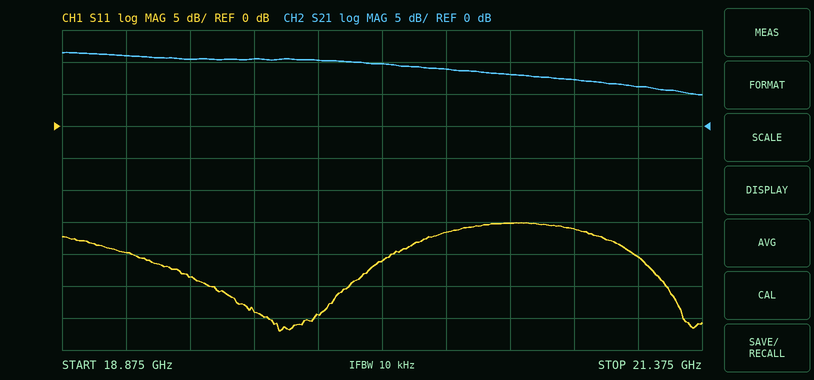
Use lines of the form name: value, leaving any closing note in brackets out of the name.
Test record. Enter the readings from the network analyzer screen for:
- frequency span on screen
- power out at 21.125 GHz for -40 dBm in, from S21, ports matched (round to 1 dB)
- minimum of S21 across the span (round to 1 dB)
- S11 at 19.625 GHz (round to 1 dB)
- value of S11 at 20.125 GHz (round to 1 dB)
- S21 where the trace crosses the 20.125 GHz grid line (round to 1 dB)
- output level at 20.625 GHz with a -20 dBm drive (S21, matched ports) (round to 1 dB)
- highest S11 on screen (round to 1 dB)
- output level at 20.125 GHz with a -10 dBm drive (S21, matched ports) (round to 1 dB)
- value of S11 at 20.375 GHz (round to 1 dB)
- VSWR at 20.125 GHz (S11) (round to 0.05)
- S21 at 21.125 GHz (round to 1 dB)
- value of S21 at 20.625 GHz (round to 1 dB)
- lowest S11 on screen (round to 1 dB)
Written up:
frequency span on screen: 2.5 GHz
power out at 21.125 GHz for -40 dBm in, from S21, ports matched: -34 dBm
minimum of S21 across the span: 5 dB
S11 at 19.625 GHz: -29 dB
value of S11 at 20.125 GHz: -21 dB
S21 where the trace crosses the 20.125 GHz grid line: 10 dB
output level at 20.625 GHz with a -20 dBm drive (S21, matched ports): -12 dBm
highest S11 on screen: -15 dB
output level at 20.125 GHz with a -10 dBm drive (S21, matched ports): 0 dBm
value of S11 at 20.375 GHz: -17 dB
VSWR at 20.125 GHz (S11): 1.20
S21 at 21.125 GHz: 6 dB
value of S21 at 20.625 GHz: 8 dB
lowest S11 on screen: -32 dB
